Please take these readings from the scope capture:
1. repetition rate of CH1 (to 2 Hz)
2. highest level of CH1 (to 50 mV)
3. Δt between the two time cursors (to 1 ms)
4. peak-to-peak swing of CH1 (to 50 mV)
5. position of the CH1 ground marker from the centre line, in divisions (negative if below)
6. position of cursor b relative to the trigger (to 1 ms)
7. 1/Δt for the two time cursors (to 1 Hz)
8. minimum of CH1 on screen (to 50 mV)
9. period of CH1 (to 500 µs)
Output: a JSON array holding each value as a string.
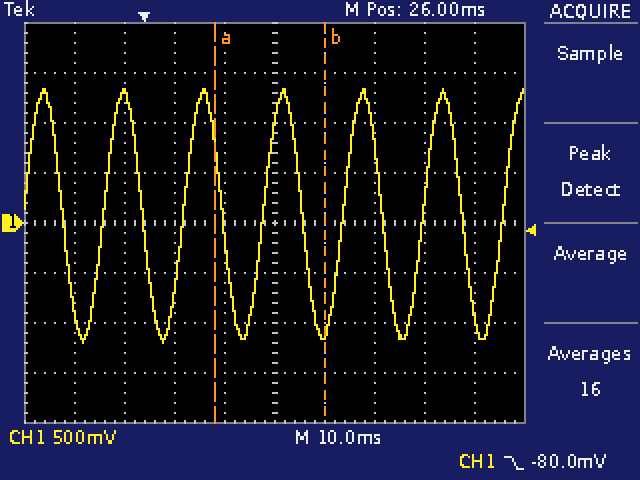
["62 Hz", "1.35 V", "22 ms", "2.55 V", "0.0 div", "+36 ms", "45 Hz", "-1.20 V", "16.0 ms"]
